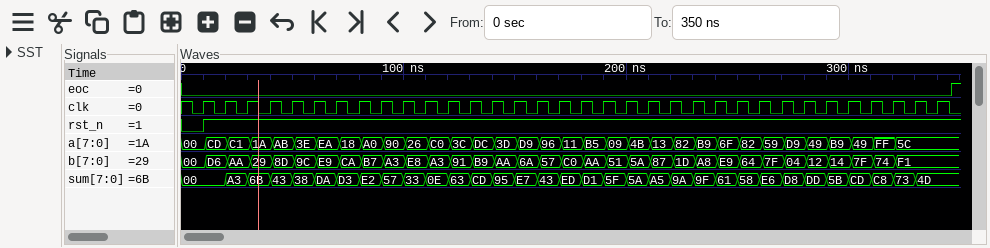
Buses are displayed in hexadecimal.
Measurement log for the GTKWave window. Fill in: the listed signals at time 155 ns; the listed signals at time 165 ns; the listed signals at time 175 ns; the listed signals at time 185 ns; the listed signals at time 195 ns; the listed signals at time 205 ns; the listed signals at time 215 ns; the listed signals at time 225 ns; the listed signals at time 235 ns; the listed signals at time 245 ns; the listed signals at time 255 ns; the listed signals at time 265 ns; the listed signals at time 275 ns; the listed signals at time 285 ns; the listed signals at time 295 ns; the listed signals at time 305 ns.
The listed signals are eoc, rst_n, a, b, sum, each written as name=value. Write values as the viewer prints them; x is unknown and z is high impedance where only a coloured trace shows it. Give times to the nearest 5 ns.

eoc=0, rst_n=1, a=D9, b=6A, sum=E7
eoc=0, rst_n=1, a=96, b=57, sum=43
eoc=0, rst_n=1, a=11, b=C0, sum=ED
eoc=0, rst_n=1, a=B5, b=AA, sum=D1
eoc=0, rst_n=1, a=09, b=51, sum=5F
eoc=0, rst_n=1, a=4B, b=5A, sum=5A
eoc=0, rst_n=1, a=13, b=87, sum=A5
eoc=0, rst_n=1, a=82, b=1D, sum=9A
eoc=0, rst_n=1, a=B9, b=A8, sum=9F
eoc=0, rst_n=1, a=6F, b=E9, sum=61
eoc=0, rst_n=1, a=82, b=64, sum=58
eoc=0, rst_n=1, a=59, b=7F, sum=E6
eoc=0, rst_n=1, a=D9, b=04, sum=D8
eoc=0, rst_n=1, a=49, b=12, sum=DD
eoc=0, rst_n=1, a=B9, b=14, sum=5B
eoc=0, rst_n=1, a=49, b=7F, sum=CD
